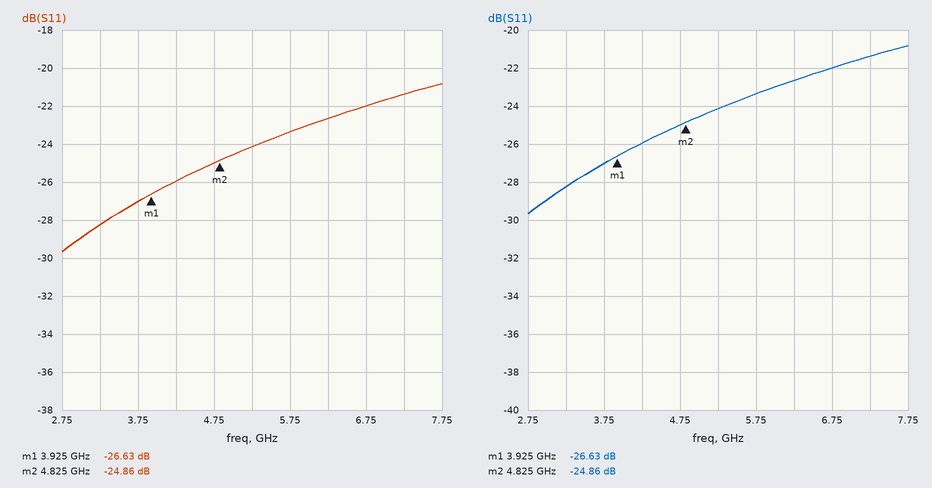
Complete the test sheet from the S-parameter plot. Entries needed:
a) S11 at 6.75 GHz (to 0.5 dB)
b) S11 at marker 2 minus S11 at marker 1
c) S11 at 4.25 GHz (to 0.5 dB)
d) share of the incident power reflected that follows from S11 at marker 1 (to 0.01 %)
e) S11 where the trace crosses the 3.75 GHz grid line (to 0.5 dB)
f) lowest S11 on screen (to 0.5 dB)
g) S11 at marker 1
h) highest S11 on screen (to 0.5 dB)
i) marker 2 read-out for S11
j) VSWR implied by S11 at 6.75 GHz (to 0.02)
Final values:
-22.0 dB
1.77 dB
-26.0 dB
0.22 %
-27.0 dB
-29.5 dB
-26.63 dB
-21.0 dB
-24.86 dB
1.18
